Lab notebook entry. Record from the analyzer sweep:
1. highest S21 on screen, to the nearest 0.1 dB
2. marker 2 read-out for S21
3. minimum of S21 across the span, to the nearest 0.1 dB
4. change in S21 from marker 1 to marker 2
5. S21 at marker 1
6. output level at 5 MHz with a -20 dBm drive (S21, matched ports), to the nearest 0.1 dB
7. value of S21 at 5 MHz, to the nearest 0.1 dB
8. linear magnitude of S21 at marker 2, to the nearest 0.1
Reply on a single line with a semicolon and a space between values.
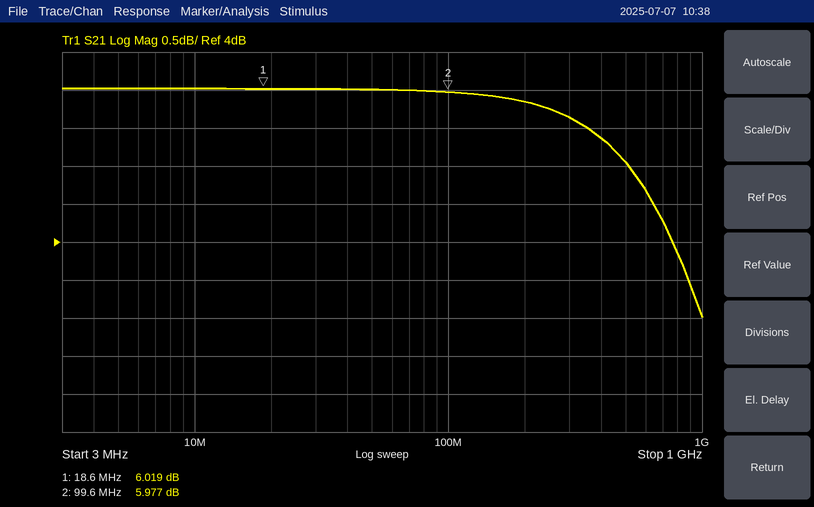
6.0 dB; 5.977 dB; 3.0 dB; -0.042 dB; 6.019 dB; -14.0 dBm; 6.0 dB; 2.0
